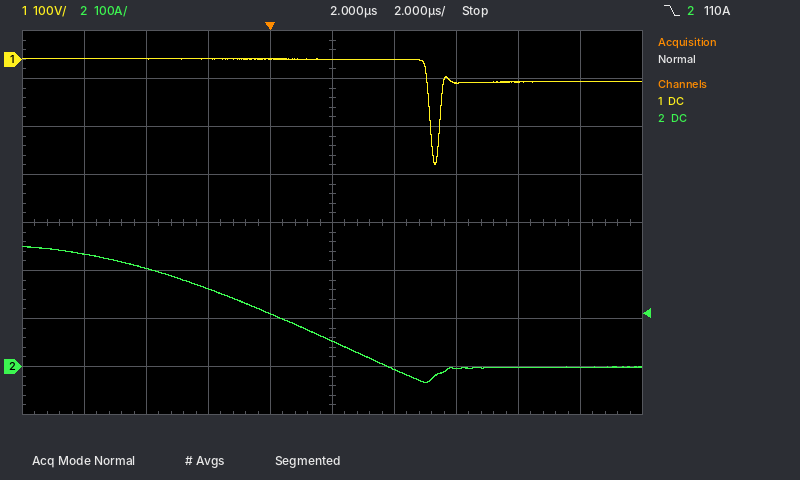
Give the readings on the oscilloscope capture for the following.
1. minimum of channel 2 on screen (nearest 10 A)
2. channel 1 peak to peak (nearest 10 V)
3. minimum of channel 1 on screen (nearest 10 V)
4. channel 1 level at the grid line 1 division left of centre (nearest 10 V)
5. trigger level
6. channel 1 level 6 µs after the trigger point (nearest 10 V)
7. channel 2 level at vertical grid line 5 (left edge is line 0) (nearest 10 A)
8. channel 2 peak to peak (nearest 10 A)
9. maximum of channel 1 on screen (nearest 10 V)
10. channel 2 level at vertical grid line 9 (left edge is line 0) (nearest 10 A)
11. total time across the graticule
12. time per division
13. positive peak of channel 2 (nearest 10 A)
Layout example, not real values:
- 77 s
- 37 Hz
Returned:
- -30 A
- 220 V
- -220 V
- 0 V
- 110 A
- -50 V
- 50 A
- 280 A
- 0 V
- 0 A
- 20 µs
- 2 µs
- 250 A
